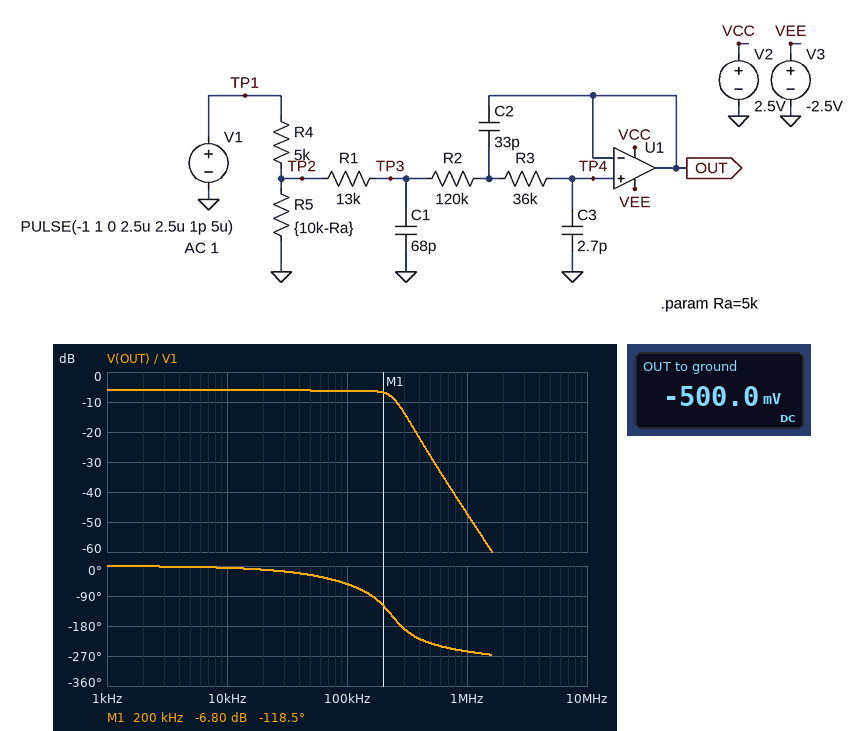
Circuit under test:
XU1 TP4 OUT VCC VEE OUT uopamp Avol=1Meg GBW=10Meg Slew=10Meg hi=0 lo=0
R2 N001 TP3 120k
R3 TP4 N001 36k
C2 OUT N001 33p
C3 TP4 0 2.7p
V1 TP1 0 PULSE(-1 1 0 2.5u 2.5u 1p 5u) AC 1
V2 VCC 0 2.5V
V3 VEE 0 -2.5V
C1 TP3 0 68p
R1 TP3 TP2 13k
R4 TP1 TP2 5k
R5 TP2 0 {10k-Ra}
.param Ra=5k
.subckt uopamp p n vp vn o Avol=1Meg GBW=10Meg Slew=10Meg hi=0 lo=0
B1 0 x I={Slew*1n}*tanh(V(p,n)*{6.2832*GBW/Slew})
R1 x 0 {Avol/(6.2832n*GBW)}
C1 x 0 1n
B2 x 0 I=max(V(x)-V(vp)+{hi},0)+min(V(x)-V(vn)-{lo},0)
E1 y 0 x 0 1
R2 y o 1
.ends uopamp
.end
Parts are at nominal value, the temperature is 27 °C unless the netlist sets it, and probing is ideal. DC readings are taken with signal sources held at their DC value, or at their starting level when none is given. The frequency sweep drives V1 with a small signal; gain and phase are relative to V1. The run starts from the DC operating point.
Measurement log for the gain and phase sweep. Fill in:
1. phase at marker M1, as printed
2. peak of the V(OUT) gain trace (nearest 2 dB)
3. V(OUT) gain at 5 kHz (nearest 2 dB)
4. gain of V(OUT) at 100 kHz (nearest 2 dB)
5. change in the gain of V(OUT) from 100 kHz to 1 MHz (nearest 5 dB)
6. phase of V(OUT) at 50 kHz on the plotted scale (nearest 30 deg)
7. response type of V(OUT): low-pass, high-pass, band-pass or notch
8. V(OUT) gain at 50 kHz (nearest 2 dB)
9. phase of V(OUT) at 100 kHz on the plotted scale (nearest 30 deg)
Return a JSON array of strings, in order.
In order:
["-118.5 deg", "-6 dB", "-6 dB", "-6 dB", "-40 dB", "-30 deg", "low-pass", "-6 dB", "-60 deg"]
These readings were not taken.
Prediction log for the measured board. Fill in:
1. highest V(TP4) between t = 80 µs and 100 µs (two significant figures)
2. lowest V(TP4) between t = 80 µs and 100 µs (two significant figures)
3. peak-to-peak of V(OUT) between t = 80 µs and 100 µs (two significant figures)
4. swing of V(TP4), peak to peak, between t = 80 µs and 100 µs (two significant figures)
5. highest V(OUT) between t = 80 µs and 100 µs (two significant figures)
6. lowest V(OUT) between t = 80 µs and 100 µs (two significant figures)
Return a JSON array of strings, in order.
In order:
["370 mV", "-370 mV", "740 mV", "740 mV", "370 mV", "-370 mV"]
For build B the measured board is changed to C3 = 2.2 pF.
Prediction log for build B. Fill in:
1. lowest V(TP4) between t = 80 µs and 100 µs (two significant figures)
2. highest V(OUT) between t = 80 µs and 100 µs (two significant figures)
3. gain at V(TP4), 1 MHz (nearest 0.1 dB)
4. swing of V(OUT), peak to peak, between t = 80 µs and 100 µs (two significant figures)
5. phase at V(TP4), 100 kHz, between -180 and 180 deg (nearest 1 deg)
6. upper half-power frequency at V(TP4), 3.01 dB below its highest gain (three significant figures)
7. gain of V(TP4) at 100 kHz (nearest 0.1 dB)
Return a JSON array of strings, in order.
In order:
["-390 mV", "390 mV", "-45.5 dB", "780 mV", "-49 deg", "274 kHz", "-6.5 dB"]
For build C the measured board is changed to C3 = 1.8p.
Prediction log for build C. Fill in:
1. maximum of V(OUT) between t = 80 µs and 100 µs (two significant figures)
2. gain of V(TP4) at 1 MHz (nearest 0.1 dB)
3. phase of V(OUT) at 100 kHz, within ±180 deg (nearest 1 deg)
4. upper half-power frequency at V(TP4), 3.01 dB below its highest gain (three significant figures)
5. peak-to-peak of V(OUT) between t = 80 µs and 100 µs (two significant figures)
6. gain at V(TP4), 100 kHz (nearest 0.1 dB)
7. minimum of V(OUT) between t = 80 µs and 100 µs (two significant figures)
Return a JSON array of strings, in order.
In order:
["390 mV", "-44.0 dB", "-47 deg", "302 kHz", "780 mV", "-6.6 dB", "-390 mV"]
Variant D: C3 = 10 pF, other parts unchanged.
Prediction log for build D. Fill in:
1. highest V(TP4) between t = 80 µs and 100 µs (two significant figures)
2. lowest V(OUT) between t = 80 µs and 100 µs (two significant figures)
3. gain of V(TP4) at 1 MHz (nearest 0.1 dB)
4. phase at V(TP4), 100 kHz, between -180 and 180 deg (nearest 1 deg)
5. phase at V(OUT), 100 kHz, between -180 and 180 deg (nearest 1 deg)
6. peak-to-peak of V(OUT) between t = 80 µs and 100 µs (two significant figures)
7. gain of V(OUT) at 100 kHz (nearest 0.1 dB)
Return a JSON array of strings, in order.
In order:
["95 mV", "-95 mV", "-57.9 dB", "-103 deg", "-104 deg", "190 mV", "-8.9 dB"]
